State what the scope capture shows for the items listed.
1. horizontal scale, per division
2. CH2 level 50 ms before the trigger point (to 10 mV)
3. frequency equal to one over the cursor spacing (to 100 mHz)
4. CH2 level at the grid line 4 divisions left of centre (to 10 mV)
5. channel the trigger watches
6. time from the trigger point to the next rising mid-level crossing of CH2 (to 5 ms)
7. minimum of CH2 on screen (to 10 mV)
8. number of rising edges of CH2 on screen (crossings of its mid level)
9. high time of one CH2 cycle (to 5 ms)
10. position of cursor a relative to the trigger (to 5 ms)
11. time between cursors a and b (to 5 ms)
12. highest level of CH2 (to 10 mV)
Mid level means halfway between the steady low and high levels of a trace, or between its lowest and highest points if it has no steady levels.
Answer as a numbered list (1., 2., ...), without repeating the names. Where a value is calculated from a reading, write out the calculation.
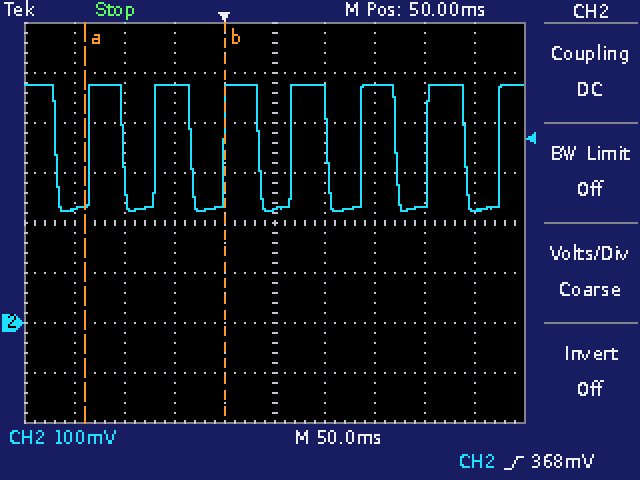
1. 50 ms
2. 480 mV
3. 1 / 140 ms ≈ 7.1 Hz
4. 230 mV
5. CH2
6. 65 ms
7. 220 mV
8. 7
9. 35 ms
10. -140 ms
11. 140 ms
12. 480 mV
